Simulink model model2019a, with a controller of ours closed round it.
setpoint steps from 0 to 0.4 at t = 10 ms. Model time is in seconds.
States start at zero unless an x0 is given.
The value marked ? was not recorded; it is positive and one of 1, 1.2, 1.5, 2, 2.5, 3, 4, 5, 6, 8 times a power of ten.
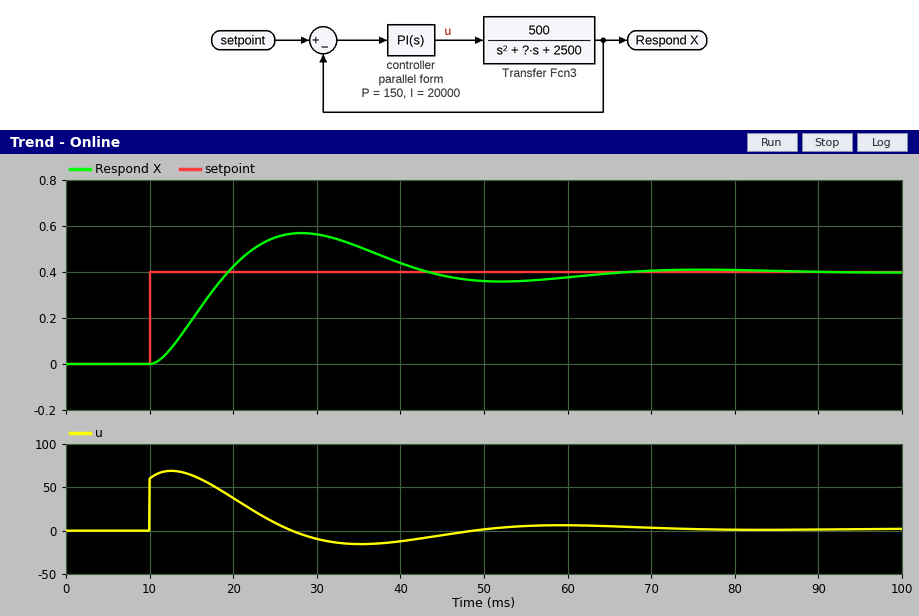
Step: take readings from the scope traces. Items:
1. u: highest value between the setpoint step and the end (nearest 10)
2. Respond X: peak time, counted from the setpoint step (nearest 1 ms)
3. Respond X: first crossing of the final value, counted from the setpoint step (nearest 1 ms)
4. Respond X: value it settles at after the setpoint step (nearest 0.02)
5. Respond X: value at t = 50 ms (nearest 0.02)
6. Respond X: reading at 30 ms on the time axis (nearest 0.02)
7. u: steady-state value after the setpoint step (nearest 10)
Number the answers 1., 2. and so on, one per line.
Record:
1. 70
2. 18 ms
3. 9 ms
4. 0.40
5. 0.36
6. 0.56
7. 0
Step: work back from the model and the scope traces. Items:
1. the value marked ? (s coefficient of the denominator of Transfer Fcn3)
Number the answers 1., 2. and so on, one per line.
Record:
1. 600
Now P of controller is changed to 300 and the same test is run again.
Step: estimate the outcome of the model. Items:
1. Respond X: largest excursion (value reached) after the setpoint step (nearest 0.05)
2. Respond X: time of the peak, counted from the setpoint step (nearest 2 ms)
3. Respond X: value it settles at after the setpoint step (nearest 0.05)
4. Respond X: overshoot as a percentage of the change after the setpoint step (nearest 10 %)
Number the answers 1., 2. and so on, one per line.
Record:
1. 0.50
2. 12 ms
3. 0.40
4. 20 %
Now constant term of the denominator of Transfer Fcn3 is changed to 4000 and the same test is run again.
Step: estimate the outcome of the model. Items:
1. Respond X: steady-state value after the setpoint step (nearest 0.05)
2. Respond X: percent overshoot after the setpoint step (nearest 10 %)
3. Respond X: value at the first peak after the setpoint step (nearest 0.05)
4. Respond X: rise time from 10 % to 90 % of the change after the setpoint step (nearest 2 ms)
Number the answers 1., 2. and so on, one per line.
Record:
1. 0.40
2. 40 %
3. 0.55
4. 6 ms
